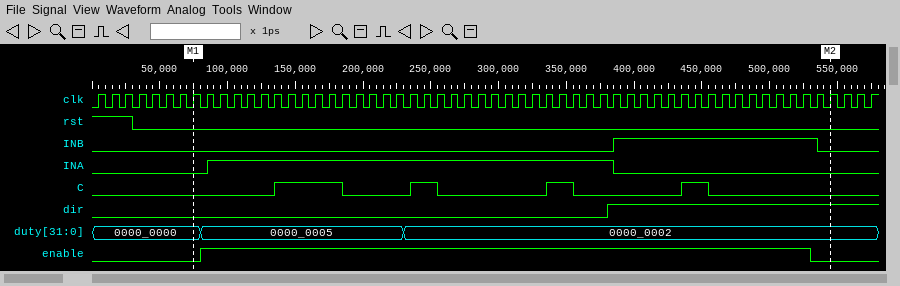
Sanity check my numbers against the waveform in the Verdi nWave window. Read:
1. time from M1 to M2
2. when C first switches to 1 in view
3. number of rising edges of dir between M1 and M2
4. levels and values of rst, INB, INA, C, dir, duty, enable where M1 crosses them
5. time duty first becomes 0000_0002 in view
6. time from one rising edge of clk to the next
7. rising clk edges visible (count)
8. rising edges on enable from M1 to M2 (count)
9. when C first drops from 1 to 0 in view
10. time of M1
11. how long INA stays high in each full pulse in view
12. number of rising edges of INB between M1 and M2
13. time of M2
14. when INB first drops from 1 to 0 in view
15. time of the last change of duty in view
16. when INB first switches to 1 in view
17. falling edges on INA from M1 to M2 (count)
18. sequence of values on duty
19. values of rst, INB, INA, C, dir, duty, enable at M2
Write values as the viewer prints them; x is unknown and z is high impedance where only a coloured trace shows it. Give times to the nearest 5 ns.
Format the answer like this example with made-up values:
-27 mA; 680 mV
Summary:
470 ns; 135 ns; 1; rst=0, INB=0, INA=0, C=0, dir=0, duty=0000_0000, enable=0; 230 ns; 10 ns; 58; 1; 185 ns; 75 ns; 300 ns; 1; 545 ns; 535 ns; 230 ns; 385 ns; 1; 0000_0000, 0000_0005, 0000_0002; rst=0, INB=0, INA=0, C=0, dir=1, duty=0000_0002, enable=0
